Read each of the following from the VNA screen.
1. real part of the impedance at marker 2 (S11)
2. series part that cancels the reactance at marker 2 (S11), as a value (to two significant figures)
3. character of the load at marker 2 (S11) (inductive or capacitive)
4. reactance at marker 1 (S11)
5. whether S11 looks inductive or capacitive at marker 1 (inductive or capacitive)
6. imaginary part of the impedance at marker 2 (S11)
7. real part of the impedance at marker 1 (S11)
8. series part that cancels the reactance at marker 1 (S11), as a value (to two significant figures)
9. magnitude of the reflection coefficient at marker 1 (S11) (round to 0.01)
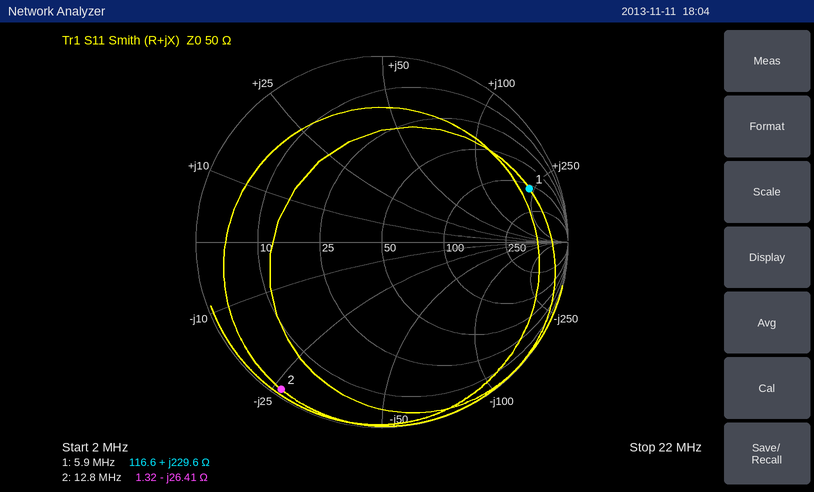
1.32 Ω
330 nH
capacitive
+229.6 Ω
inductive
-26.41 Ω
116.6 Ω
120 pF
0.84
